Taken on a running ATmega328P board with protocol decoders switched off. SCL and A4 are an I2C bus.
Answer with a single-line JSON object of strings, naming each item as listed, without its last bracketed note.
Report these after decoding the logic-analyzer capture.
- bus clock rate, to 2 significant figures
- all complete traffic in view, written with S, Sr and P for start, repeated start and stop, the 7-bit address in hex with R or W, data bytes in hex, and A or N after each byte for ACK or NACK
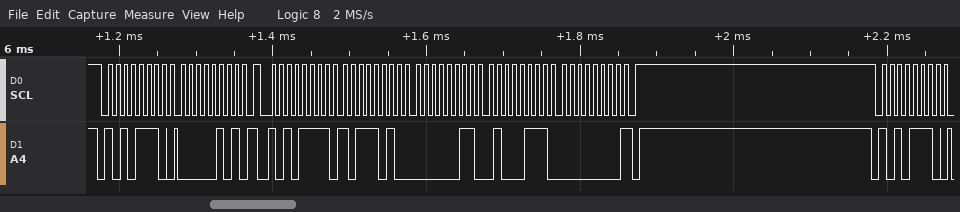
{"bus clock rate, to 2 significant figures": "100 kHz", "all complete traffic in view, written with S, Sr and P for start, repeated start and stop, the 7-bit address in hex with R or W, data bytes in hex, and A or N after each byte for ACK or NACK": "S 57W A 05 A Sr 57R A BA A 03 A 47 A 00 N P S 57W A"}
